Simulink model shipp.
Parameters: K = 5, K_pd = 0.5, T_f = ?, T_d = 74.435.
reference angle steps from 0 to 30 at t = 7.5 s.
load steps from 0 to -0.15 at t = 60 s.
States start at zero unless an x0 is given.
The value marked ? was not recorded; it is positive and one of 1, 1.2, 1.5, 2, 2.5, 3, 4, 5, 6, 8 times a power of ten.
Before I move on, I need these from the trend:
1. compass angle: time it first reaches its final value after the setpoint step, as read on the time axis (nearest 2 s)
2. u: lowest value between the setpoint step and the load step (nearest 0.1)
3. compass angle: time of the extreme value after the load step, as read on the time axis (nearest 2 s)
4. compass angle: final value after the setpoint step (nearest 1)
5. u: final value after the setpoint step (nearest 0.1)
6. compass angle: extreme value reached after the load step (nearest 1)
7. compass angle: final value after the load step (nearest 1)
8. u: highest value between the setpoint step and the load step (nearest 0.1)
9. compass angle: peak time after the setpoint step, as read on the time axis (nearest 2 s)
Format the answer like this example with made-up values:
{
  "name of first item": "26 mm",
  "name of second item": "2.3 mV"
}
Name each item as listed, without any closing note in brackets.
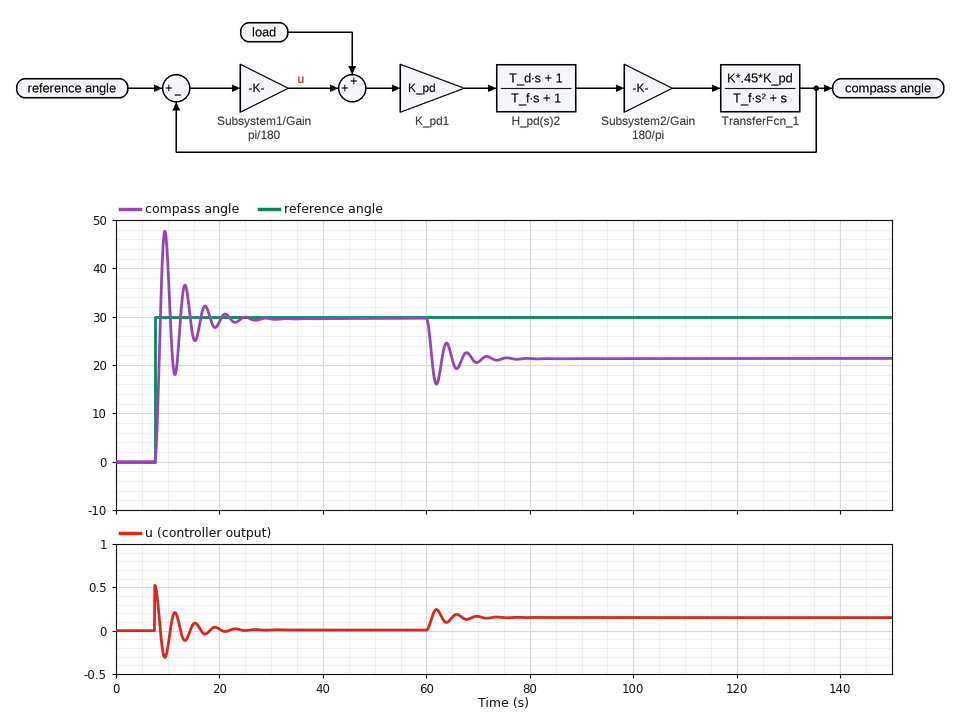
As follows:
{
  "compass angle: time it first reaches its final value after the setpoint step, as read on the time axis": "8 s",
  "u: lowest value between the setpoint step and the load step": "-0.3",
  "compass angle: time of the extreme value after the load step, as read on the time axis": "62 s",
  "compass angle: final value after the setpoint step": "30",
  "u: final value after the setpoint step": "0.0",
  "compass angle: extreme value reached after the load step": "16",
  "compass angle: final value after the load step": "21",
  "u: highest value between the setpoint step and the load step": "0.5",
  "compass angle: peak time after the setpoint step, as read on the time axis": "10 s"
}
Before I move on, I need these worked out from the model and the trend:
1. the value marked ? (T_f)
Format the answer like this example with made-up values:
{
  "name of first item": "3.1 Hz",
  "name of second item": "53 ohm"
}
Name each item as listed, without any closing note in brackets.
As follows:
{
  "the value marked ?": "4"
}
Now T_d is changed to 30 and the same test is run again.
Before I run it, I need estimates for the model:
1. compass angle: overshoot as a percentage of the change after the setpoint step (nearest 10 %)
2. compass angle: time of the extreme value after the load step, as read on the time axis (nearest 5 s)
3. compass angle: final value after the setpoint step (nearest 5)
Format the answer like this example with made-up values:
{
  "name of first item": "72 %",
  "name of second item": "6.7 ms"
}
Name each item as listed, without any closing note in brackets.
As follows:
{
  "compass angle: overshoot as a percentage of the change after the setpoint step": "40 %",
  "compass angle: time of the extreme value after the load step, as read on the time axis": "65 s",
  "compass angle: final value after the setpoint step": "30"
}
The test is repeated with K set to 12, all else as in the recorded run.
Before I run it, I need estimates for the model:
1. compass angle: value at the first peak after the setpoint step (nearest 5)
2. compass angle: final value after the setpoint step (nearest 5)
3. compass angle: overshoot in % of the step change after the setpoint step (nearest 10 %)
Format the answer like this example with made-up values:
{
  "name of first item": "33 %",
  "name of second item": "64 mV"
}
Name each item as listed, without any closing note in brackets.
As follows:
{
  "compass angle: value at the first peak after the setpoint step": "50",
  "compass angle: final value after the setpoint step": "30",
  "compass angle: overshoot in % of the step change after the setpoint step": "70 %"
}
